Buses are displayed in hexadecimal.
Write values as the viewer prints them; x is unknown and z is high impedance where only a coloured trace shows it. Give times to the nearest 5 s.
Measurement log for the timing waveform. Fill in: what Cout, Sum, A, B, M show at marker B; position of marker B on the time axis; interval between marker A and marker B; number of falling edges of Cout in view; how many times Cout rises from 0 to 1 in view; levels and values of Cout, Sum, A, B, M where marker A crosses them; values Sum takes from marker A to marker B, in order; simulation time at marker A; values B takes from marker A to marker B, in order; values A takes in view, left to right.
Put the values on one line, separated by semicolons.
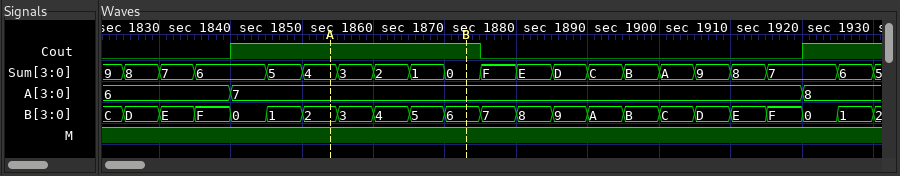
Cout=1, Sum=0, A=7, B=6, M=1; 1875 s; 20 s; 1; 2; Cout=1, Sum=4, A=7, B=2, M=1; 4, 3, 2, 1, 0; 1855 s; 2, 3, 4, 5, 6; 6, 7, 8
